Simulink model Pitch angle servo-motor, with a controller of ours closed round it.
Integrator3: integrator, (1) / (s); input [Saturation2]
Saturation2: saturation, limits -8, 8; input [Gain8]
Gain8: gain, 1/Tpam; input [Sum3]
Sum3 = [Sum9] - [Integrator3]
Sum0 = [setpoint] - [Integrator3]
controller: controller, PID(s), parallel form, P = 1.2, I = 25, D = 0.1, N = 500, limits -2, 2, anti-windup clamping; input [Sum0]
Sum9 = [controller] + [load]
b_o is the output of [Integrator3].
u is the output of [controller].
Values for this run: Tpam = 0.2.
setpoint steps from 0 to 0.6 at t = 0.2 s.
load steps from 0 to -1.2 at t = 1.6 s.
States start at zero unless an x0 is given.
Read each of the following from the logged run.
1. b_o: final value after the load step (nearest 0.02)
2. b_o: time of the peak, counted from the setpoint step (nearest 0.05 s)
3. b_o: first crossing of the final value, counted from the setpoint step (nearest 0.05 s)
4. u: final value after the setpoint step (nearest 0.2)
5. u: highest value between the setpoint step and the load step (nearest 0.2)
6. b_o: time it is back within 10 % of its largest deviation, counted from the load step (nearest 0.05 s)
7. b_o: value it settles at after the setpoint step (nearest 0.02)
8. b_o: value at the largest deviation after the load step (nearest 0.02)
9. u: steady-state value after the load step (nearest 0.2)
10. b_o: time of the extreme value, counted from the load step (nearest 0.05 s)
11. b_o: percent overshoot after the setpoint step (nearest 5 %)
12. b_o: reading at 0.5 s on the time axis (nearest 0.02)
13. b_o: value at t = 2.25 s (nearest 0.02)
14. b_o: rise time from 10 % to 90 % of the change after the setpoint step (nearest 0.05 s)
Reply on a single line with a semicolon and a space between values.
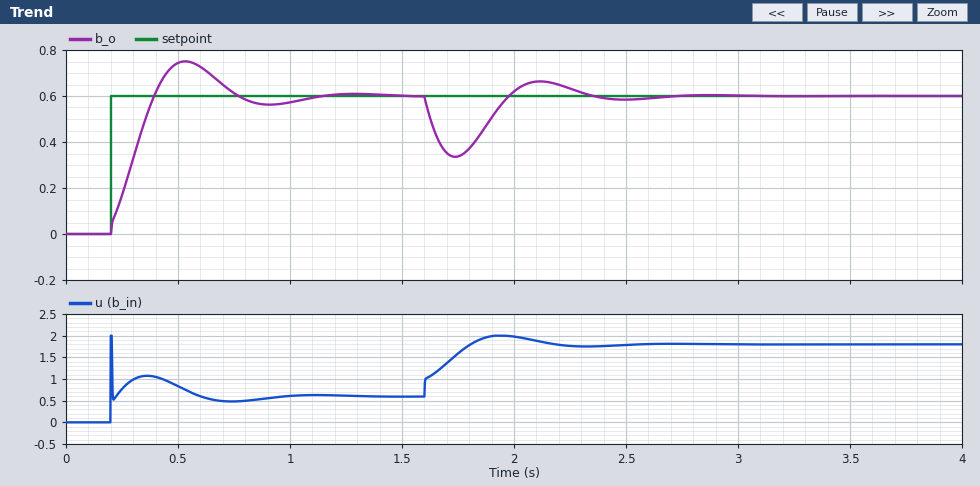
0.60; 0.35 s; 0.20 s; 0.6; 2.0; 0.65 s; 0.60; 0.34; 1.8; 0.15 s; 25 %; 0.74; 0.64; 0.15 s
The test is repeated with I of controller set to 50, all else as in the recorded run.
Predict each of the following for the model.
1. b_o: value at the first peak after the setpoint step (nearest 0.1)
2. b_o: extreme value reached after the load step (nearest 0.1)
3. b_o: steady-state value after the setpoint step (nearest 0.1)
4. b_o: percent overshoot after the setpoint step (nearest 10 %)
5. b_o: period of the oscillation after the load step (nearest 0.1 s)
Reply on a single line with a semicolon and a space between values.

0.8; 0.4; 0.6; 40 %; 0.5 s
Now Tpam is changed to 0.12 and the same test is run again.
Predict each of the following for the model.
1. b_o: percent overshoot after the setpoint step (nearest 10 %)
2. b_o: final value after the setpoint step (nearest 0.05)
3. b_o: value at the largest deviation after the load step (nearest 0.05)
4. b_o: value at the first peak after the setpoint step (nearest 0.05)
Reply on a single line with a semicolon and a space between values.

20 %; 0.60; 0.30; 0.70
